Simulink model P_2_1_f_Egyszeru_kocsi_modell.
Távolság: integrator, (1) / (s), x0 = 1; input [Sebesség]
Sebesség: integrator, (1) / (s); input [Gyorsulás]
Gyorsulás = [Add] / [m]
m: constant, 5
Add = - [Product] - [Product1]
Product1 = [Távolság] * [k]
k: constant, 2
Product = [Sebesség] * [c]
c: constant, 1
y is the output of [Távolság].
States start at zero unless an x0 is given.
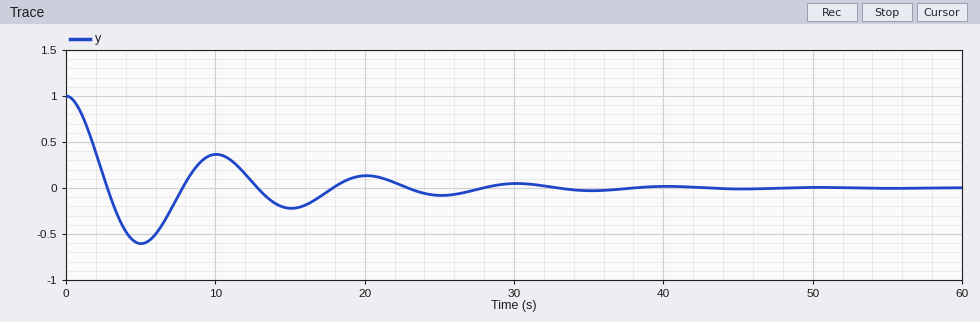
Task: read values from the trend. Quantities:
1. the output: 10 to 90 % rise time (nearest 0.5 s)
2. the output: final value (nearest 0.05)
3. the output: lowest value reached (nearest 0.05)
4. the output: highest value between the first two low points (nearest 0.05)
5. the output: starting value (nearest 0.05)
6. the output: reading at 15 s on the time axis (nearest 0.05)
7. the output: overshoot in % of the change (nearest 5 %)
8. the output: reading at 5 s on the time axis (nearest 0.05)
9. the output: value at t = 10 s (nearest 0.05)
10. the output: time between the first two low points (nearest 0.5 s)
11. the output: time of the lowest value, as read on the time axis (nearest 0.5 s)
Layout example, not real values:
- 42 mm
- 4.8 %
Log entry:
- 2.0 s
- 0.00
- -0.60
- 0.35
- 1.00
- -0.20
- 60 %
- -0.60
- 0.35
- 10.0 s
- 5.0 s
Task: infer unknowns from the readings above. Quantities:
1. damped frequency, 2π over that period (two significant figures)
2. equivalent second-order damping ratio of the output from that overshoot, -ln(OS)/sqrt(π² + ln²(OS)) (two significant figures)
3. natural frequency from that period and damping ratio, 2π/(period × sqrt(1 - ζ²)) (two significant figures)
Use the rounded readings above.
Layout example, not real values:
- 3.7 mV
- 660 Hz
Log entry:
- 0.63 rad/s
- 0.16
- 0.64 rad/s
